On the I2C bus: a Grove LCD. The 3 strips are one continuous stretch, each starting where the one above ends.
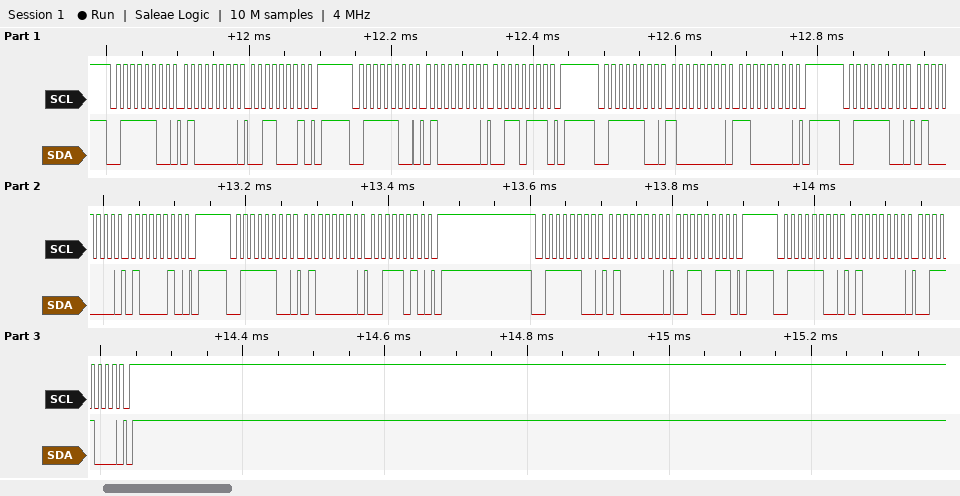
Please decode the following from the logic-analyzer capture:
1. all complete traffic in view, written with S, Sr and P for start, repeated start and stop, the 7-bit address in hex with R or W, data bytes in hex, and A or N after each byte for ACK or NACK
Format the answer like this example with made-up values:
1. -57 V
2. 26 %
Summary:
1. S 3EW A 40 A 31 A P S 3EW A 40 A 37 A P S 3EW A 80 A C0 A P S 3EW A 40 A 42 A P S 3EW A 40 A 3A A P S 3EW A 40 A 33 A P S 3EW A 40 A 38 A P
